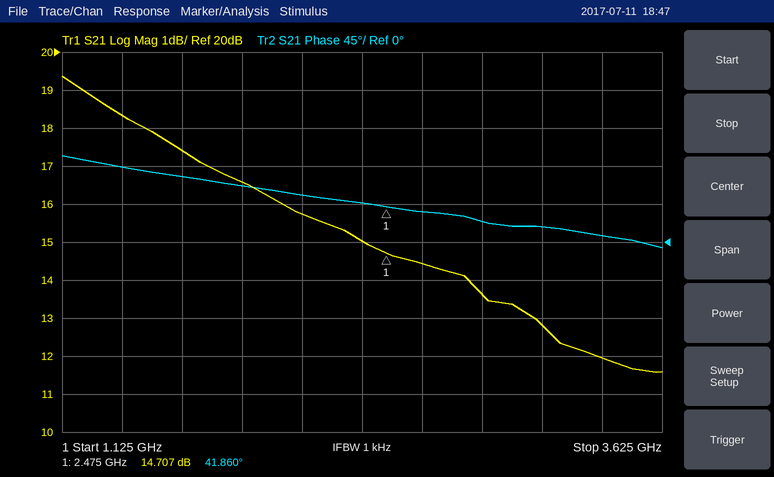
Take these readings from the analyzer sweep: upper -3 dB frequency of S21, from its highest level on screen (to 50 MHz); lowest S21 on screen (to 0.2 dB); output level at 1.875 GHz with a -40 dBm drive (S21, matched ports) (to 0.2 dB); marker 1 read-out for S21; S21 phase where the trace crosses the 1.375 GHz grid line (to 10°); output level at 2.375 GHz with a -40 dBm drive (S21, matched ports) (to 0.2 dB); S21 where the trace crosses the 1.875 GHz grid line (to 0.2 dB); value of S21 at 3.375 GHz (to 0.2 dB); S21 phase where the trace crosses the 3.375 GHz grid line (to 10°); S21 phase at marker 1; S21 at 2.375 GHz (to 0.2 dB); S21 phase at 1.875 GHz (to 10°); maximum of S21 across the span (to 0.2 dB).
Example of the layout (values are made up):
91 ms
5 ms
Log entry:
1.95 GHz
11.6 dB
-23.4 dBm
14.707 dB
90°
-25.0 dBm
16.6 dB
12.0 dB
10°
41.860°
15.0 dB
70°
19.4 dB
